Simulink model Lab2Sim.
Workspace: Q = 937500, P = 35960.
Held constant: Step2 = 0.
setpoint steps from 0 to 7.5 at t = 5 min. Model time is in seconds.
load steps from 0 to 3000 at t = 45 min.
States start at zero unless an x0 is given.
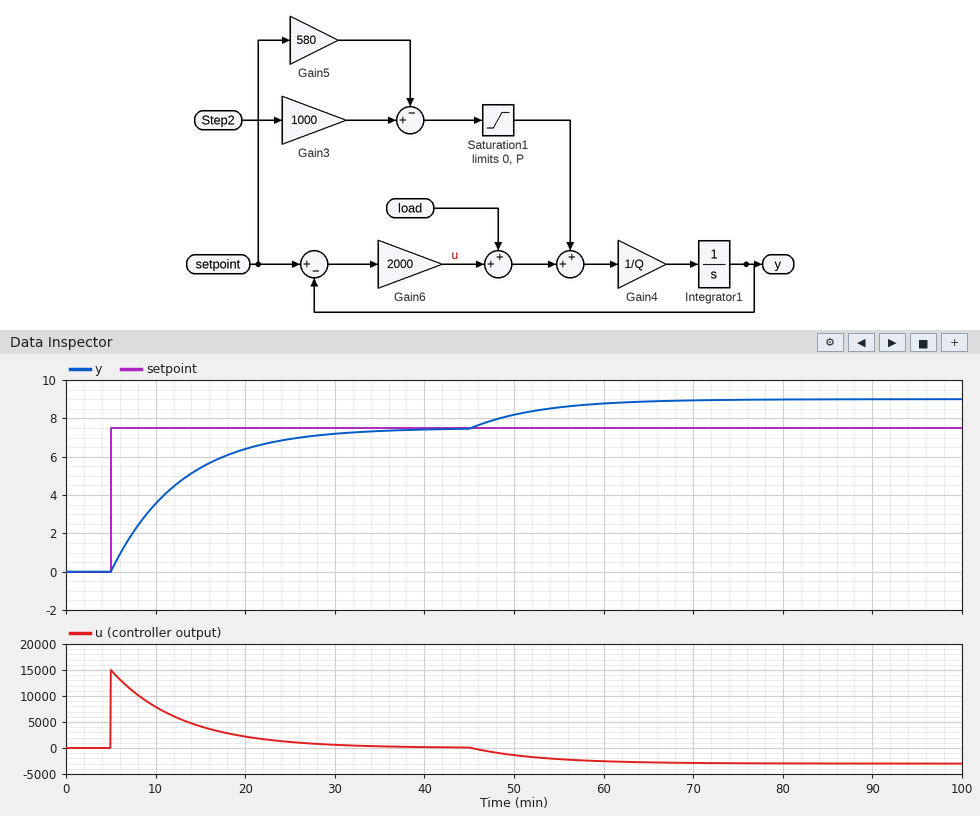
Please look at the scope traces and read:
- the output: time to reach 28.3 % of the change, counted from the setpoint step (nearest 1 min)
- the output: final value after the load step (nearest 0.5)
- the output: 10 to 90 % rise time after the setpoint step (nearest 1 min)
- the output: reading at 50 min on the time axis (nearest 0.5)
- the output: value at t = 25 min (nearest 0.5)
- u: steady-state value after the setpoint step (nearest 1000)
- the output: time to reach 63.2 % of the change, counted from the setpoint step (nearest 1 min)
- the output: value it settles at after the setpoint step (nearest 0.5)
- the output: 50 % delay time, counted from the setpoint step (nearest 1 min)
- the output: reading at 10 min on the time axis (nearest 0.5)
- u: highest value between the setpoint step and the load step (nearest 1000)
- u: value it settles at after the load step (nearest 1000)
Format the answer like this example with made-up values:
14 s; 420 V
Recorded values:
3 min; 9.0; 17 min; 8.0; 7.0; 0; 8 min; 7.5; 5 min; 3.5; 15000; -3000
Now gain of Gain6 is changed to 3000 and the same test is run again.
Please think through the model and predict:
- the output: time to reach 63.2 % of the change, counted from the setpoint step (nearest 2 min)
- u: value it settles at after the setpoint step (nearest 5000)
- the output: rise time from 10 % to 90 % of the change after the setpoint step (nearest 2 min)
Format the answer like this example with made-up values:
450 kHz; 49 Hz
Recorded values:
6 min; 0; 12 min
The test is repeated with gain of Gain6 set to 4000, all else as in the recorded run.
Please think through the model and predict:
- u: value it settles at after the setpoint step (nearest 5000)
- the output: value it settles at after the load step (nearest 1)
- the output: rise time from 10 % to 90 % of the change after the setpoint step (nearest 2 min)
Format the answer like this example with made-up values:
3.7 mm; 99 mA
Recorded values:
0; 8; 8 min
